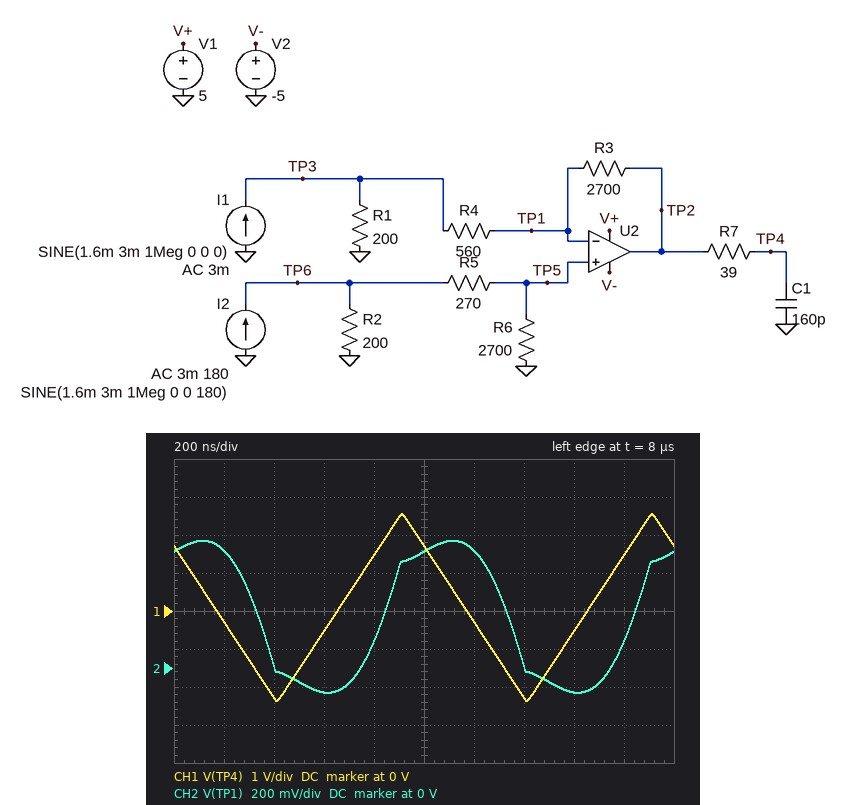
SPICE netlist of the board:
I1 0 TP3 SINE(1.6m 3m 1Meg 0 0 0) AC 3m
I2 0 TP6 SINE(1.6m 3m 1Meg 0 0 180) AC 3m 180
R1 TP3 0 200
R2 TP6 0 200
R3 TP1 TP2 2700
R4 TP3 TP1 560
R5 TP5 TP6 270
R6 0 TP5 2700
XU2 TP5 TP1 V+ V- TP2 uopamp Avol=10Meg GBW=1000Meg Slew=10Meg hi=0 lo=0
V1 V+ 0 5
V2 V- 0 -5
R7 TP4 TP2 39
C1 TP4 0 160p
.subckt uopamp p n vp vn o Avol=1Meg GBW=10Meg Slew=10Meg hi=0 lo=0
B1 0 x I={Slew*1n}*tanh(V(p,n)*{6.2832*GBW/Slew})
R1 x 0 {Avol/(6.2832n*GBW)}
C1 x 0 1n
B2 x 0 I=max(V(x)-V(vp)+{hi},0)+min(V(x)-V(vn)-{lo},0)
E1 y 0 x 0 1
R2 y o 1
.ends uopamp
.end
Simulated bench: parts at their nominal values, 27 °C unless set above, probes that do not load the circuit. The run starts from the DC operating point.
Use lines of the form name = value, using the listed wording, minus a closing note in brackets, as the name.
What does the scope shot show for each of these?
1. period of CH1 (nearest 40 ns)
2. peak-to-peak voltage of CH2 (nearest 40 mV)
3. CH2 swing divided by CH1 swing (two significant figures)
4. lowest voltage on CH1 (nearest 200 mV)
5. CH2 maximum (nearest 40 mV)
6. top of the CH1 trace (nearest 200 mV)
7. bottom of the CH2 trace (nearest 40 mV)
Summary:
period of CH1 = 1.00 µs
peak-to-peak voltage of CH2 = 800 mV
CH2 swing divided by CH1 swing = 0.16
lowest voltage on CH1 = -2.4 V
CH2 maximum = 680 mV
top of the CH1 trace = 2.6 V
bottom of the CH2 trace = -120 mV
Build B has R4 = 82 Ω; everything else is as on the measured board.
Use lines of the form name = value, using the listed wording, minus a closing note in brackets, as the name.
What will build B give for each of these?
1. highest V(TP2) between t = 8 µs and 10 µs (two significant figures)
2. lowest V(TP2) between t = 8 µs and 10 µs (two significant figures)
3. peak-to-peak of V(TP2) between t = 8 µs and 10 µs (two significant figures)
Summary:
highest V(TP2) between t = 8 µs and 10 µs = 2.3 V
lowest V(TP2) between t = 8 µs and 10 µs = -2.7 V
peak-to-peak of V(TP2) between t = 8 µs and 10 µs = 5.0 V
